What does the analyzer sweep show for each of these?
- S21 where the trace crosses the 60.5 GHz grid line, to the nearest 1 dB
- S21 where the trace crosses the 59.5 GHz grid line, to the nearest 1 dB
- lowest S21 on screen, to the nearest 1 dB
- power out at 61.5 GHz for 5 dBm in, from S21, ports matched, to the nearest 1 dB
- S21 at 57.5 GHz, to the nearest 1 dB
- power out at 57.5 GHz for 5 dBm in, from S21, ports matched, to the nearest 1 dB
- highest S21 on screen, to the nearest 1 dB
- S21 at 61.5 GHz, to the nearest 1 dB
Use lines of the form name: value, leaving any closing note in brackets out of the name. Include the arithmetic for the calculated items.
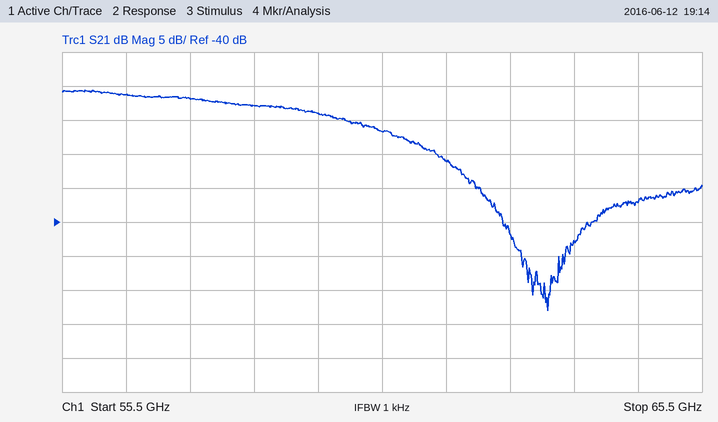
S21 where the trace crosses the 60.5 GHz grid line, to the nearest 1 dB: -27 dB
S21 where the trace crosses the 59.5 GHz grid line, to the nearest 1 dB: -24 dB
lowest S21 on screen, to the nearest 1 dB: -53 dB
power out at 61.5 GHz for 5 dBm in, from S21, ports matched, to the nearest 1 dB: 5 dBm + (-31 dB) = -26 dBm
S21 at 57.5 GHz, to the nearest 1 dB: -22 dB
power out at 57.5 GHz for 5 dBm in, from S21, ports matched, to the nearest 1 dB: 5 dBm + (-22 dB) = -17 dBm
highest S21 on screen, to the nearest 1 dB: -21 dB
S21 at 61.5 GHz, to the nearest 1 dB: -31 dB
